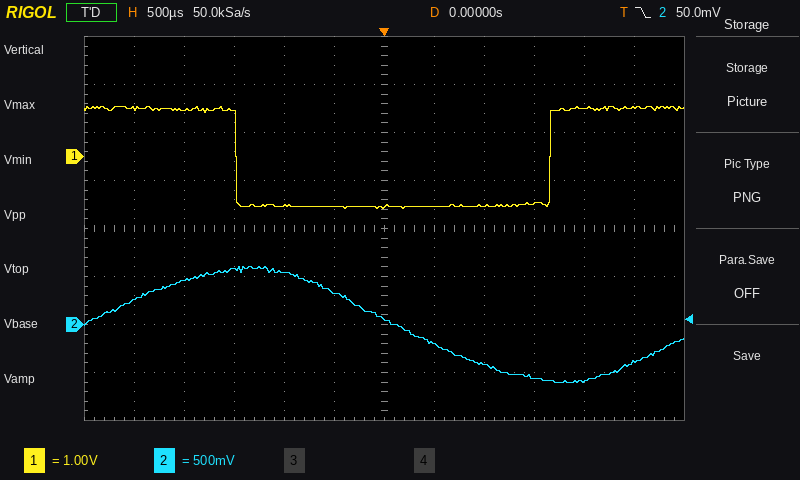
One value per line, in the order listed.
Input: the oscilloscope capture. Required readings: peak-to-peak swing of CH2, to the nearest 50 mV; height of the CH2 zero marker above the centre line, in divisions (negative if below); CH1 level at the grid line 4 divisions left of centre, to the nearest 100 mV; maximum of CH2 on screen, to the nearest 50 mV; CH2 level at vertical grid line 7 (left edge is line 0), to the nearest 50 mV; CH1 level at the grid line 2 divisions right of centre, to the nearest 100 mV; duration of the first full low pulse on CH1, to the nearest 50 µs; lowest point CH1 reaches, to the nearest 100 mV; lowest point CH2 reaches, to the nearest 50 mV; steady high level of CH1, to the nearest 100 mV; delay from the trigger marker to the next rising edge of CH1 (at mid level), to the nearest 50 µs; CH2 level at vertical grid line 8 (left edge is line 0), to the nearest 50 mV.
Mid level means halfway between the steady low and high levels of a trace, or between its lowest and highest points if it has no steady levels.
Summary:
1.20 V
-2.0 div
1.0 V
600 mV
-200 mV
-1.0 V
3.15 ms
-1.1 V
-600 mV
1.0 V
1.65 ms
-400 mV
